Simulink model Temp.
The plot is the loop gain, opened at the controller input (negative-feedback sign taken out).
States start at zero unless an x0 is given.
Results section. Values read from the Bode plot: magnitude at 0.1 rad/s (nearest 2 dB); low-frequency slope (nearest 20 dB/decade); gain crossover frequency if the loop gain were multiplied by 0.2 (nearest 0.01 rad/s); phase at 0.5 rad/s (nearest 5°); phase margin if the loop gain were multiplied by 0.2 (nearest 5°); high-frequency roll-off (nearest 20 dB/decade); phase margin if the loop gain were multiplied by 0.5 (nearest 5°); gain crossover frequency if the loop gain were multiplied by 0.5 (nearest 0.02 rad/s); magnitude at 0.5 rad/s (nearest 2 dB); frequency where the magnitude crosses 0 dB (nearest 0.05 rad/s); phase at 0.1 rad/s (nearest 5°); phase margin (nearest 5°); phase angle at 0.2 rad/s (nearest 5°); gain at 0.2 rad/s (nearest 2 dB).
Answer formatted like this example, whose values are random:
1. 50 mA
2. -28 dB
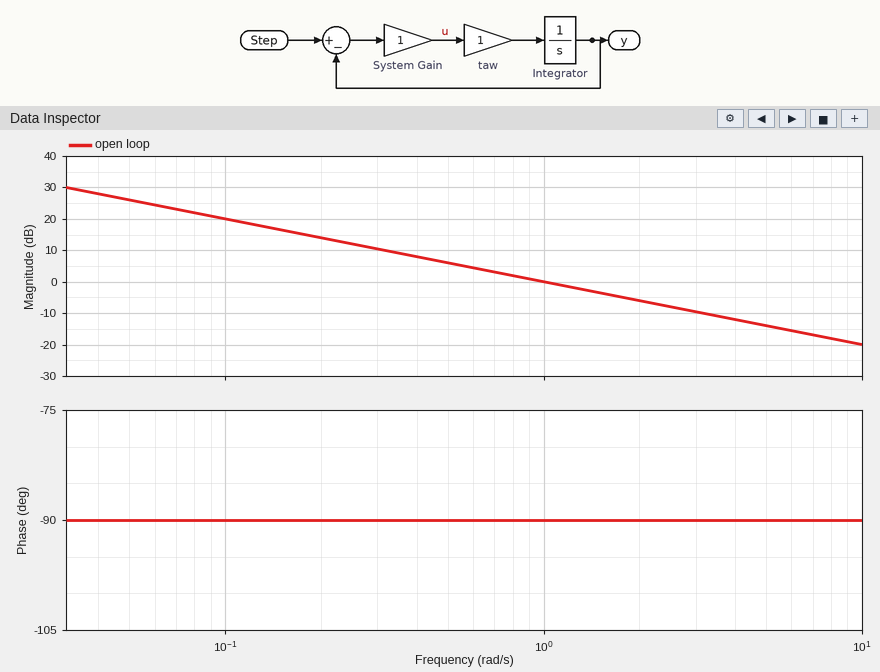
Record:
1. 20 dB
2. -20 dB/decade
3. 0.20 rad/s
4. -90°
5. 90°
6. -20 dB/decade
7. 90°
8. 0.50 rad/s
9. 6 dB
10. 1.00 rad/s
11. -90°
12. 90°
13. -90°
14. 14 dB
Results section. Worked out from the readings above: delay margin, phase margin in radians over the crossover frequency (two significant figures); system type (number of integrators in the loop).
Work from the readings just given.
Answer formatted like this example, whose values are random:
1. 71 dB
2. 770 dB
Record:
1. 1.6 s
2. 1
